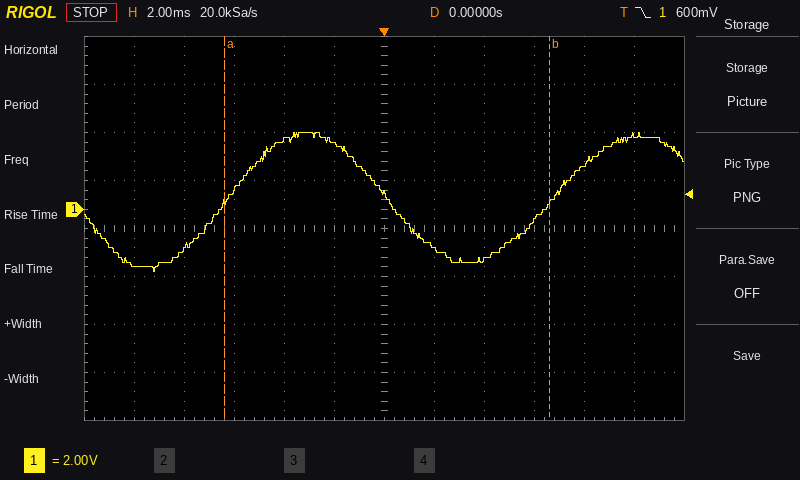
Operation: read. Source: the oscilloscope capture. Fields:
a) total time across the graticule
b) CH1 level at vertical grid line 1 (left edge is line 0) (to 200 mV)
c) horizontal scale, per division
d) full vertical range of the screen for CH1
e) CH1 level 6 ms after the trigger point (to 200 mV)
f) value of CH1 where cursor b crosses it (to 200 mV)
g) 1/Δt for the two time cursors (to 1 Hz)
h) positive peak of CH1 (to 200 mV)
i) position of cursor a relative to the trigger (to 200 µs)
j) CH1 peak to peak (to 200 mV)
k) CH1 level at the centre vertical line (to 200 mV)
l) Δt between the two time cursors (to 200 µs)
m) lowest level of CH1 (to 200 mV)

24 ms
-2.4 V
2 ms
16 V
-400 mV
200 mV
77 Hz
3.2 V
-6.4 ms
5.8 V
600 mV
13.0 ms
-2.6 V
